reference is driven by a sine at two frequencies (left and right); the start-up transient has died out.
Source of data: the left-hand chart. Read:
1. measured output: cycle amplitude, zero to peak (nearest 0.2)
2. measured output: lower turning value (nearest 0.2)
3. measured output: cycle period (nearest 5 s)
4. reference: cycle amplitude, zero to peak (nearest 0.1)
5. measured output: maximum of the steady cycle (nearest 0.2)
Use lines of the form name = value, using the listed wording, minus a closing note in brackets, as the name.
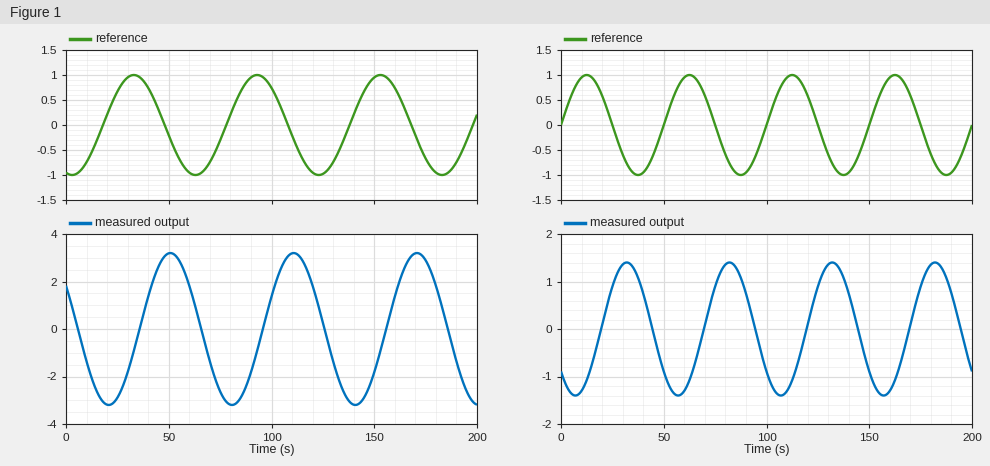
measured output: cycle amplitude, zero to peak = 3.2
measured output: lower turning value = -3.2
measured output: cycle period = 60 s
reference: cycle amplitude, zero to peak = 1.0
measured output: maximum of the steady cycle = 3.2
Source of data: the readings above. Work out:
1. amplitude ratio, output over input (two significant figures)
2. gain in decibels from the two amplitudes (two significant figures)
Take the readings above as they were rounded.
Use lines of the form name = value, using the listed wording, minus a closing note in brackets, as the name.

amplitude ratio, output over input = 3.2
gain in decibels from the two amplitudes = 10 dB
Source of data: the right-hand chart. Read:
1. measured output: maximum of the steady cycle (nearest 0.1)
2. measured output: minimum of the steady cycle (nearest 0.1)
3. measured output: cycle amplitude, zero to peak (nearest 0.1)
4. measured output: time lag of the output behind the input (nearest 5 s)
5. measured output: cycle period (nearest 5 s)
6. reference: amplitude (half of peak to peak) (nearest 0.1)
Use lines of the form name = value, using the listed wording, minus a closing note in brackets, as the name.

measured output: maximum of the steady cycle = 1.4
measured output: minimum of the steady cycle = -1.4
measured output: cycle amplitude, zero to peak = 1.4
measured output: time lag of the output behind the input = 20 s
measured output: cycle period = 50 s
reference: amplitude (half of peak to peak) = 1.0
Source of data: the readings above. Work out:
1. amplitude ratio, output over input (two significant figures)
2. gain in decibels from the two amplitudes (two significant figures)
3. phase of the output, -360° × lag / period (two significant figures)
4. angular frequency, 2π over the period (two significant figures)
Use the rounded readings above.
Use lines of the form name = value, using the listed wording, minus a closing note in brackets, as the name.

amplitude ratio, output over input = 1.4
gain in decibels from the two amplitudes = 2.9 dB
phase of the output, -360° × lag / period = -140°
angular frequency, 2π over the period = 0.13 rad/s
